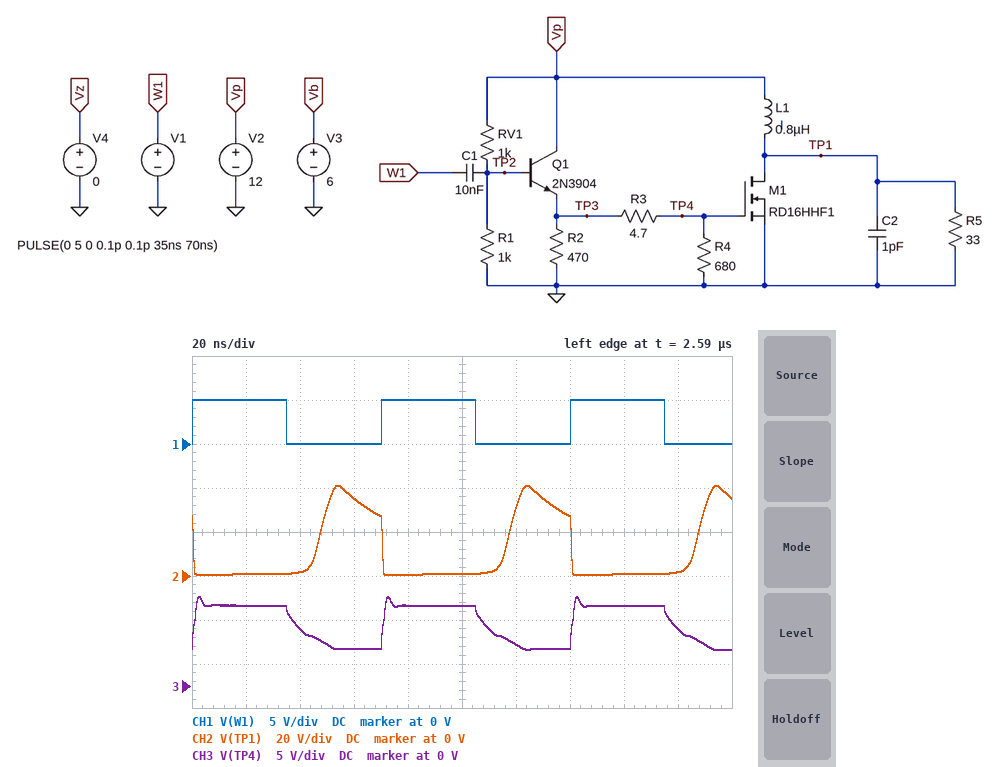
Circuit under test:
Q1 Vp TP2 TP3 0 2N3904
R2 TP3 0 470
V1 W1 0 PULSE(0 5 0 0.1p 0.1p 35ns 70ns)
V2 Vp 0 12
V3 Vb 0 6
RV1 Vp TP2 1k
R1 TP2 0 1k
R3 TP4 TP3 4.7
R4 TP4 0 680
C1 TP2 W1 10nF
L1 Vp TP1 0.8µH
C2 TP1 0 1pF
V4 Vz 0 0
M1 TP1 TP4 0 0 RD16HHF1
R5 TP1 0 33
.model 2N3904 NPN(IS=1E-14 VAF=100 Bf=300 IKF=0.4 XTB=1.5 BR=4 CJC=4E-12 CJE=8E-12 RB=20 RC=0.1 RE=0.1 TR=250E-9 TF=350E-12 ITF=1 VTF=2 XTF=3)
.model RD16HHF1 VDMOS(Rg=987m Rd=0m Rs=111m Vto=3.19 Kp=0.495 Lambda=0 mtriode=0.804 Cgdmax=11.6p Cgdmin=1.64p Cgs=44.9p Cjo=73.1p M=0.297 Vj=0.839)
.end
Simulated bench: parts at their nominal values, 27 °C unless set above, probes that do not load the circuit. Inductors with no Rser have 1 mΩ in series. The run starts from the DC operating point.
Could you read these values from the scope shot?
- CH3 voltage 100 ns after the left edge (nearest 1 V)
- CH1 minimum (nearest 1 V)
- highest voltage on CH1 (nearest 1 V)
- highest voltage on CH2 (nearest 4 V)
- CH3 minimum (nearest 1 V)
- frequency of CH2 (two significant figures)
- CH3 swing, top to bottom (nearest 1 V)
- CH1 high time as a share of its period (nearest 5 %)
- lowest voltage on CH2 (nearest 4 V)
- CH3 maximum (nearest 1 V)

9 V
0 V
5 V
40 V
4 V
14 MHz
6 V
50 %
0 V
10 V
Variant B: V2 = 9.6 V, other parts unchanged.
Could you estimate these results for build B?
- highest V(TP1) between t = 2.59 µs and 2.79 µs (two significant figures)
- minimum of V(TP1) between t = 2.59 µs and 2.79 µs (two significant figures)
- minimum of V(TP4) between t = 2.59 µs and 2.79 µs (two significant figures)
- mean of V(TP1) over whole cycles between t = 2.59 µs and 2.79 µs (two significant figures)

31 V
350 mV
2.9 V
9.6 V
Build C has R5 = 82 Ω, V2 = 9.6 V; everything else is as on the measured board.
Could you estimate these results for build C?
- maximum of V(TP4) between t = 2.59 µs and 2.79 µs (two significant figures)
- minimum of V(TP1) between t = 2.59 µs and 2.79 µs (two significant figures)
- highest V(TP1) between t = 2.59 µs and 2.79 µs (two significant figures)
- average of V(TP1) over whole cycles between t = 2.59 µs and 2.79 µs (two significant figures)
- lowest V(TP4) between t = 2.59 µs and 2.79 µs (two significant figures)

8.9 V
100 mV
39 V
9.6 V
2.9 V
